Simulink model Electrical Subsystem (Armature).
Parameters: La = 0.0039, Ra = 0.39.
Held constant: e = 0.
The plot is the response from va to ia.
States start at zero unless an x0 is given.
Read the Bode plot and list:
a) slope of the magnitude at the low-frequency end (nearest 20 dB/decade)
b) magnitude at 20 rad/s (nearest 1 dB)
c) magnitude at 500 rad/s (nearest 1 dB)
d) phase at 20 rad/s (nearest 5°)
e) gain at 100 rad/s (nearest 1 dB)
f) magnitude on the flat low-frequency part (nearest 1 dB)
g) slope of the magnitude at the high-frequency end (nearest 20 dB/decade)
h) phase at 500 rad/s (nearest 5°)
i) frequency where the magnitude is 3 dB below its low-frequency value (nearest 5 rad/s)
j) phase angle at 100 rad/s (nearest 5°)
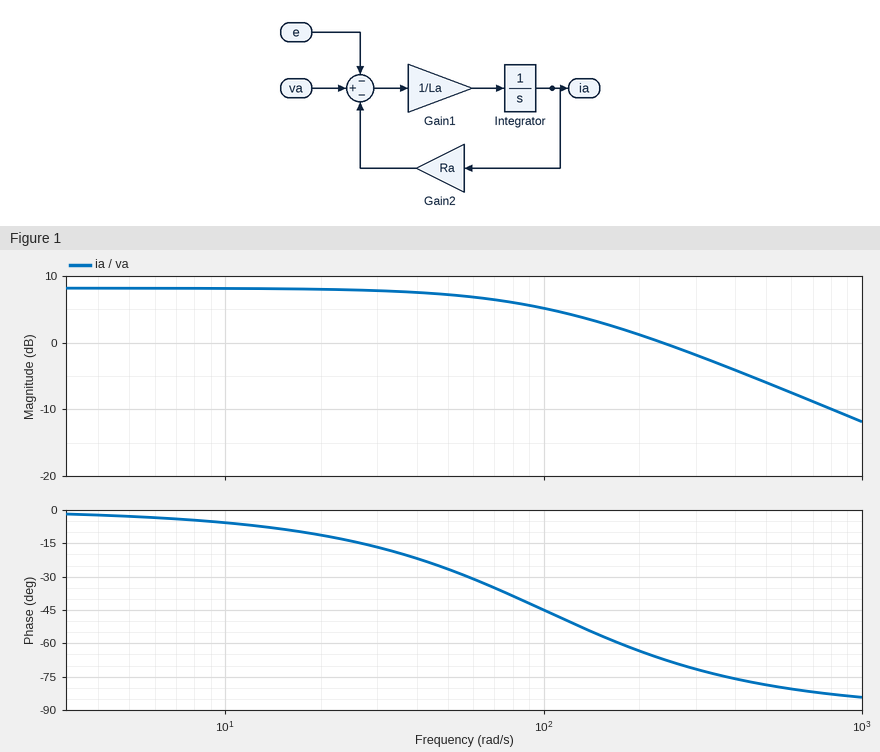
0 dB/decade
8 dB
-6 dB
-10°
5 dB
8 dB
-20 dB/decade
-80°
100 rad/s
-45°
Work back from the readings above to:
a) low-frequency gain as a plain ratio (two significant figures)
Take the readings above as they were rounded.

2.5
